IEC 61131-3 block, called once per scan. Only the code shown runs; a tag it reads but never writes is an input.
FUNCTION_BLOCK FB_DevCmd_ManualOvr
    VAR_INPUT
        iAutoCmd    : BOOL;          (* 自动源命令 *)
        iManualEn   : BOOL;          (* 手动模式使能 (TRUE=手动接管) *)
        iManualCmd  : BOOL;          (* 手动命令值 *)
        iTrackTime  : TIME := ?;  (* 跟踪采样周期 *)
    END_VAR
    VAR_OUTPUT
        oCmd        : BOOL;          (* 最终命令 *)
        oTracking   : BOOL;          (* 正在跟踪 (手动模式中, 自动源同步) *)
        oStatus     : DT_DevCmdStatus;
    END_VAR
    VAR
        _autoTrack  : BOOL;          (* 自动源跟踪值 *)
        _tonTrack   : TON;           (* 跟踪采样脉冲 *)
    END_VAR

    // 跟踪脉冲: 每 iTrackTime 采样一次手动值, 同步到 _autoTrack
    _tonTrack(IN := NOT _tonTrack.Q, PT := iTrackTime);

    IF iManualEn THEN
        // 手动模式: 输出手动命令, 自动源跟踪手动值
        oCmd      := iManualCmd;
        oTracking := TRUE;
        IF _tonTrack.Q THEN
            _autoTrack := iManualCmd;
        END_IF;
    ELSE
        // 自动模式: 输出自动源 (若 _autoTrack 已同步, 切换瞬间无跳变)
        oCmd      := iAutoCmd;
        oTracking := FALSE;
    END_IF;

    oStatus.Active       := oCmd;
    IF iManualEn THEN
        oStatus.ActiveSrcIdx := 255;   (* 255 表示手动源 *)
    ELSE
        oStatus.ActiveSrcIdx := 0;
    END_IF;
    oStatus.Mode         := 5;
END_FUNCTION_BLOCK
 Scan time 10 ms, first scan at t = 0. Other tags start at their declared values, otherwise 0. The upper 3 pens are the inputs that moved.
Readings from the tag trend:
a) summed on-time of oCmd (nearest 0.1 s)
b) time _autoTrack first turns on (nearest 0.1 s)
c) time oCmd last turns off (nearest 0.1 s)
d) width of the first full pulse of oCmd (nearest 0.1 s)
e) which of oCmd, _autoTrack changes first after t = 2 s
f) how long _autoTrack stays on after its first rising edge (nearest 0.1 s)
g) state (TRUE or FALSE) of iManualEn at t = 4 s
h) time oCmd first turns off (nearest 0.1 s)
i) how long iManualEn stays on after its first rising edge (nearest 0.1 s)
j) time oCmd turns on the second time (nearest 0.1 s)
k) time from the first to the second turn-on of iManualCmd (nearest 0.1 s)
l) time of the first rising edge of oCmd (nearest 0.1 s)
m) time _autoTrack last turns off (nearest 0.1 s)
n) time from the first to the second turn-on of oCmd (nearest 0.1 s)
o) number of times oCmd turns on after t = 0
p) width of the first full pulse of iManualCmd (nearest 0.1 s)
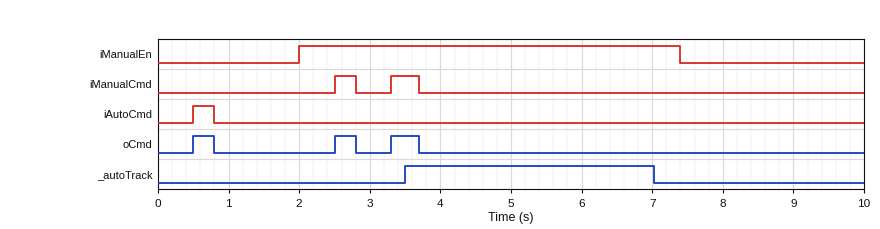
1.0 s
3.5 s
3.7 s
0.3 s
oCmd
3.5 s
TRUE
0.8 s
5.4 s
2.5 s
0.8 s
0.5 s
7.0 s
2.0 s
3
0.3 s
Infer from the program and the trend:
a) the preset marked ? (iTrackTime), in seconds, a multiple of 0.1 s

3.5 s
